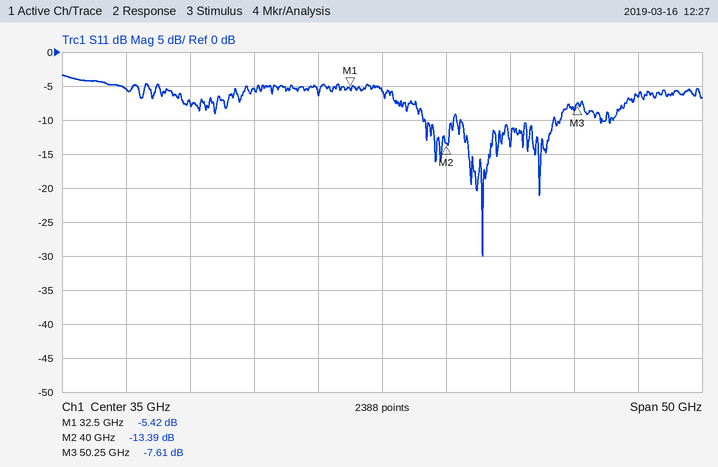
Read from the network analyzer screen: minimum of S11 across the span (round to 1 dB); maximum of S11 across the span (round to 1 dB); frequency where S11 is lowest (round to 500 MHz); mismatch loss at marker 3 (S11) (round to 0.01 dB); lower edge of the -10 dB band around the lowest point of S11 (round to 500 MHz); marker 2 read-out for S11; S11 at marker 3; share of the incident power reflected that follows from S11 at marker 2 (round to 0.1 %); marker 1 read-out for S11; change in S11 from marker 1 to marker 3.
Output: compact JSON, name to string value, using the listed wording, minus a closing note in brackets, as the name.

{"minimum of S11 across the span": "-30 dB", "maximum of S11 across the span": "-3 dB", "frequency where S11 is lowest": "43.0 GHz", "mismatch loss at marker 3 (S11)": "0.83 dB", "lower edge of the -10 dB band around the lowest point of S11": "41.0 GHz", "marker 2 read-out for S11": "-13.39 dB", "S11 at marker 3": "-7.61 dB", "share of the incident power reflected that follows from S11 at marker 2": "4.6 %", "marker 1 read-out for S11": "-5.42 dB", "change in S11 from marker 1 to marker 3": "-2.19 dB"}
